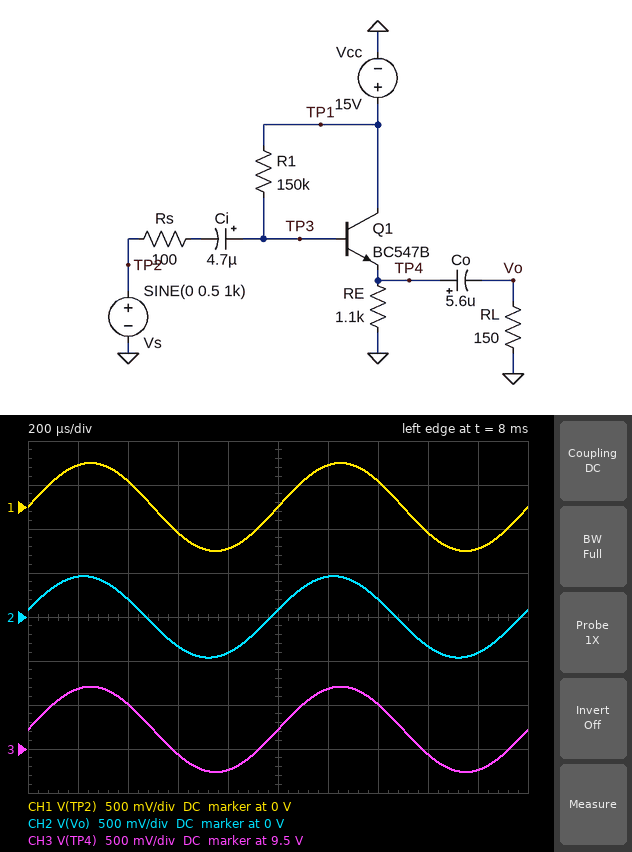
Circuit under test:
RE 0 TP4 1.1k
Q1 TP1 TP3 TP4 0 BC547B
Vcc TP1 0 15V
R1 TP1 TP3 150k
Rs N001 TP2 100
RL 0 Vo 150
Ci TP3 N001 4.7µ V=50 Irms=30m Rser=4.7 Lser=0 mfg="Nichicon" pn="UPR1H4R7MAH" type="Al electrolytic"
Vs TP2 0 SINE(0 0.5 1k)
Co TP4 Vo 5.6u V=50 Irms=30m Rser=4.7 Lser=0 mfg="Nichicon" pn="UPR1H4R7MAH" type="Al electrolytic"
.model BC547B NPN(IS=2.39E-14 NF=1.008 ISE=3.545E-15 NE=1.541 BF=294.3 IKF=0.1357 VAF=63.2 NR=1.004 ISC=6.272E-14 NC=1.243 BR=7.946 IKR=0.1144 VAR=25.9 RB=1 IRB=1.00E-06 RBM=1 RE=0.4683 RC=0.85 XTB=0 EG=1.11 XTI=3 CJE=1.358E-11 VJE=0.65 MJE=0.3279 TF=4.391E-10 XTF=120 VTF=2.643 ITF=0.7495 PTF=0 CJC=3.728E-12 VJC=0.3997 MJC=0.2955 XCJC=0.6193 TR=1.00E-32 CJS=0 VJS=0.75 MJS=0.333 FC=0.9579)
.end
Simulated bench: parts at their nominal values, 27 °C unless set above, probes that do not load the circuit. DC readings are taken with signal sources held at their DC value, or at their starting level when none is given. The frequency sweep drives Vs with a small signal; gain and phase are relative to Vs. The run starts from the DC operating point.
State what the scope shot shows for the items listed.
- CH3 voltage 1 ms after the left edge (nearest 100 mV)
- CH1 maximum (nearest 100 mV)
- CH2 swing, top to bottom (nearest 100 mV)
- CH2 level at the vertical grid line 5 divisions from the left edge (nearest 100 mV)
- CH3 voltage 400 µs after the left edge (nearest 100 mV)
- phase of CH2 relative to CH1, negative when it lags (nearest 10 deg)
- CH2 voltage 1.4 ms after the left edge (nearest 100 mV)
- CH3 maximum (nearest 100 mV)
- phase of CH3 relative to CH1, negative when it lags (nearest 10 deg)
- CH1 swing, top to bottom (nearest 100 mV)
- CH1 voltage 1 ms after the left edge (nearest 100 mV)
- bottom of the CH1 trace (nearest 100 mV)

9.7 V
500 mV
900 mV
100 mV
10.0 V
10 deg
200 mV
10.2 V
0 deg
1.0 V
0 V
-500 mV
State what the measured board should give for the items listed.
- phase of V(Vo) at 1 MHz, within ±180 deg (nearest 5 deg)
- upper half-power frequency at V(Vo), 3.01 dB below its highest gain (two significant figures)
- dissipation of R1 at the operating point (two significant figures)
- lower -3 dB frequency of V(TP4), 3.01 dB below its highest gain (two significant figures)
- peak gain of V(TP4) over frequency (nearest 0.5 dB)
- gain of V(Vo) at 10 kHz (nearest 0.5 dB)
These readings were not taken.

0 deg
190 MHz
140 µW
350 mHz
0 dB
-0.5 dB
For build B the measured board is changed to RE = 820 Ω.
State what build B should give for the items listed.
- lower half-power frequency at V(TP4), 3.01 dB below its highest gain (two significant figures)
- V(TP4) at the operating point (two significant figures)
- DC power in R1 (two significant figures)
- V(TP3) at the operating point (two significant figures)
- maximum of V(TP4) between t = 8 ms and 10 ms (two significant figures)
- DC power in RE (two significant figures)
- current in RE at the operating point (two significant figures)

390 mHz
8.8 V
200 µW
9.5 V
9.3 V
94 mW
11 mA
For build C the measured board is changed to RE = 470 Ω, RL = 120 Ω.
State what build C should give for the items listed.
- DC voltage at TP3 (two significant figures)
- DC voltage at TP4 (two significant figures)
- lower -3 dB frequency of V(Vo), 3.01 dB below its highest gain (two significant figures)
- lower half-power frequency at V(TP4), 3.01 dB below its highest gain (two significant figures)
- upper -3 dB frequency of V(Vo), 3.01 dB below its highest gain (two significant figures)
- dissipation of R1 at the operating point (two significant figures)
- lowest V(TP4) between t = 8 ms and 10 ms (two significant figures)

7.5 V
6.8 V
220 Hz
520 mHz
160 MHz
370 µW
6.3 V
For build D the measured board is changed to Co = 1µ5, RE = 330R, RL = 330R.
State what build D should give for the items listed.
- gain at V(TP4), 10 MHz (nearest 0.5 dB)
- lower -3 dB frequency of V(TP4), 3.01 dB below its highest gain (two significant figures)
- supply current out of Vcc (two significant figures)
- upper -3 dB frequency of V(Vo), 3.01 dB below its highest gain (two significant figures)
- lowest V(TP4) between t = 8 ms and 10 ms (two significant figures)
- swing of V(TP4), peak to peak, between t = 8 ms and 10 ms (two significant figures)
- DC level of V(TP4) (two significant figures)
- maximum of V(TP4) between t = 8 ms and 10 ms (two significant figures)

0 dB
640 mHz
17 mA
260 MHz
5.1 V
980 mV
5.6 V
6.1 V
